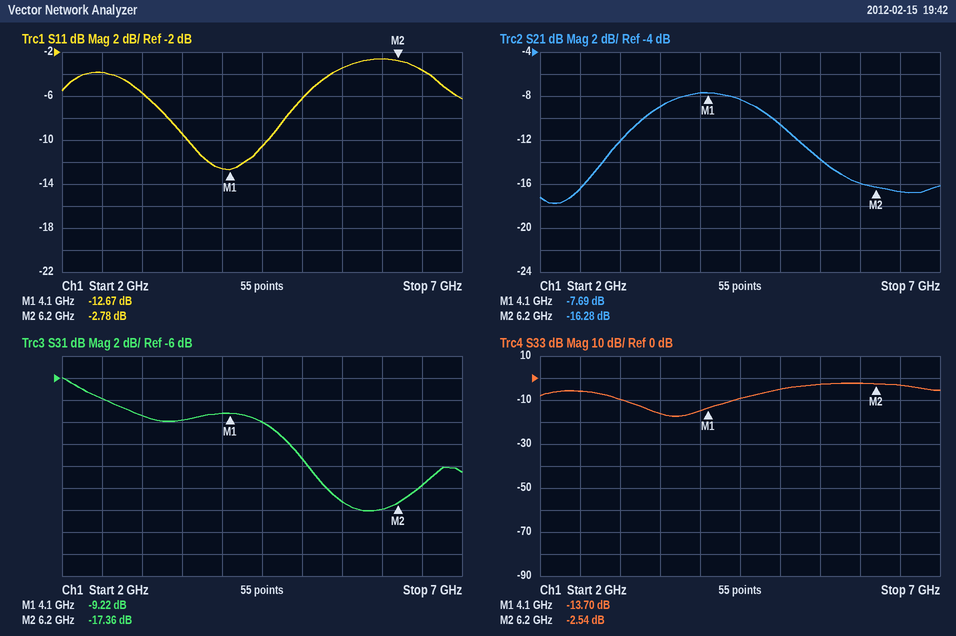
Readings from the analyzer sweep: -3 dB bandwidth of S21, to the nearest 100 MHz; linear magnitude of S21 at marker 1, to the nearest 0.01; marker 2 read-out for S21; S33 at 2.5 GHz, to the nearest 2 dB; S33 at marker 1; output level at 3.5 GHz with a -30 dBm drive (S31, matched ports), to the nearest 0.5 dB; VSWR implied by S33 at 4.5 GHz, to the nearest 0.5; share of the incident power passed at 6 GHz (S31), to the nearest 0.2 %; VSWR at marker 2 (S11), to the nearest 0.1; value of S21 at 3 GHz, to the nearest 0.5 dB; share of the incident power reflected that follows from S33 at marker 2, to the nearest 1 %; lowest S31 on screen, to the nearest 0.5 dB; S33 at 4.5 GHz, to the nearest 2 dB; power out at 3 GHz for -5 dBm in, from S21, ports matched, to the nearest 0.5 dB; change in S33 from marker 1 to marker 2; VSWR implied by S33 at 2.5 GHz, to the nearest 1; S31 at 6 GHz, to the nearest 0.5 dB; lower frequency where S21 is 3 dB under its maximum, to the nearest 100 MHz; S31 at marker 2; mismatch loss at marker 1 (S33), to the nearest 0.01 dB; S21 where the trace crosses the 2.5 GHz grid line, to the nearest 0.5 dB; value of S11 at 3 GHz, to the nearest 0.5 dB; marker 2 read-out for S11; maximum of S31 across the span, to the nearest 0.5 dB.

1.8 GHz
0.41
-16.28 dB
-6 dB
-13.70 dB
-40.0 dBm
2.0
1.6 %
6.3
-12.0 dB
56 %
-18.0 dB
-10 dB
-17.0 dBm
11.16 dB
3
-18.0 dB
3.2 GHz
-17.36 dB
0.19 dB
-16.5 dB
-5.5 dB
-2.78 dB
-6.0 dB
